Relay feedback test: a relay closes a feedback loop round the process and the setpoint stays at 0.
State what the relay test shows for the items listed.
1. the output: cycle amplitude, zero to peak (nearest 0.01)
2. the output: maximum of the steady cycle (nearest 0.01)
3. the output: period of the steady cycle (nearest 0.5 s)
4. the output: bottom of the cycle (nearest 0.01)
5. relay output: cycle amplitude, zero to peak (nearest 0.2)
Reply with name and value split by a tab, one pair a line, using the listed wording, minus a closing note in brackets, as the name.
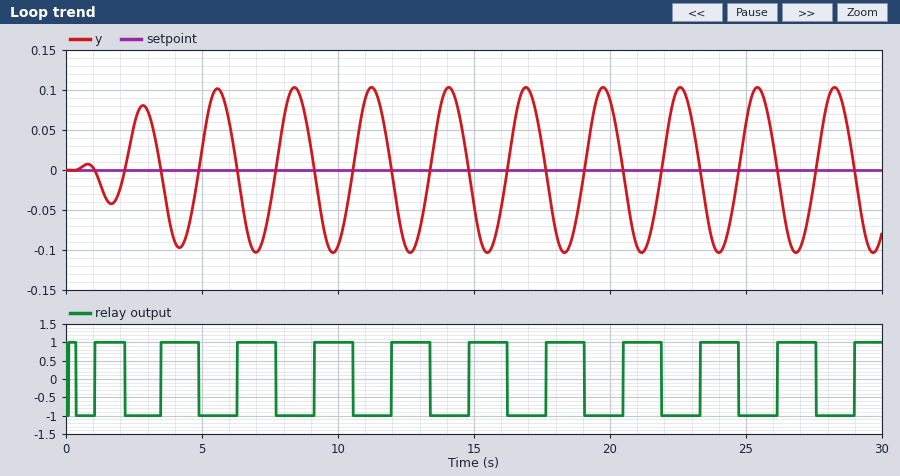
the output: cycle amplitude, zero to peak	0.10
the output: maximum of the steady cycle	0.10
the output: period of the steady cycle	3.0 s
the output: bottom of the cycle	-0.10
relay output: cycle amplitude, zero to peak	1.0
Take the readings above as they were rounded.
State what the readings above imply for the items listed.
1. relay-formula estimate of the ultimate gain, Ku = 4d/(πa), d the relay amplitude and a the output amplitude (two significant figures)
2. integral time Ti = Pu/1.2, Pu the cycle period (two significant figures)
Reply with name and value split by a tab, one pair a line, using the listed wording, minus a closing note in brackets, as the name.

relay-formula estimate of the ultimate gain, Ku = 4d/(πa), d the relay amplitude and a the output amplitude	13
integral time Ti = Pu/1.2, Pu the cycle period	2.5 s
